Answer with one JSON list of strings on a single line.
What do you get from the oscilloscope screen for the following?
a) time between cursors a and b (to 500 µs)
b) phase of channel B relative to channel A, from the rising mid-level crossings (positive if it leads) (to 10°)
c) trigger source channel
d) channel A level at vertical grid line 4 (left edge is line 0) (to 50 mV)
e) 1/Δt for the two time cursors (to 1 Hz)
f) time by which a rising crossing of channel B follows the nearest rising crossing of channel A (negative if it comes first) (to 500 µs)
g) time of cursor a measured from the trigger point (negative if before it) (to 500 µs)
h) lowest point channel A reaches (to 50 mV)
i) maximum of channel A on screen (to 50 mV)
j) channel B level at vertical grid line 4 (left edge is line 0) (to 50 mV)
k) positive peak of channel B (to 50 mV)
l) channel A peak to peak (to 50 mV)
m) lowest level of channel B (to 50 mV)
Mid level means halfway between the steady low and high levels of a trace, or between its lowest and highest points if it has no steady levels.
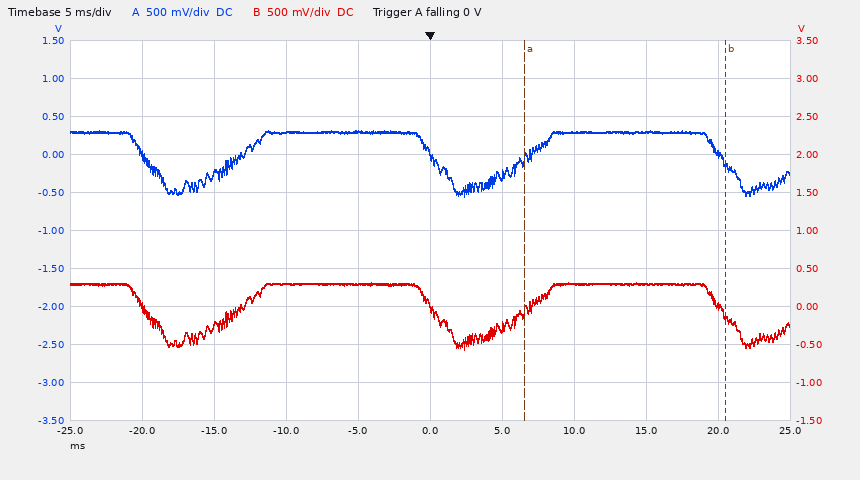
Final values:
["14.0 ms", "0°", "channel A", "300 mV", "71 Hz", "0.0 ms", "+6.5 ms", "-550 mV", "300 mV", "300 mV", "300 mV", "850 mV", "-550 mV"]
